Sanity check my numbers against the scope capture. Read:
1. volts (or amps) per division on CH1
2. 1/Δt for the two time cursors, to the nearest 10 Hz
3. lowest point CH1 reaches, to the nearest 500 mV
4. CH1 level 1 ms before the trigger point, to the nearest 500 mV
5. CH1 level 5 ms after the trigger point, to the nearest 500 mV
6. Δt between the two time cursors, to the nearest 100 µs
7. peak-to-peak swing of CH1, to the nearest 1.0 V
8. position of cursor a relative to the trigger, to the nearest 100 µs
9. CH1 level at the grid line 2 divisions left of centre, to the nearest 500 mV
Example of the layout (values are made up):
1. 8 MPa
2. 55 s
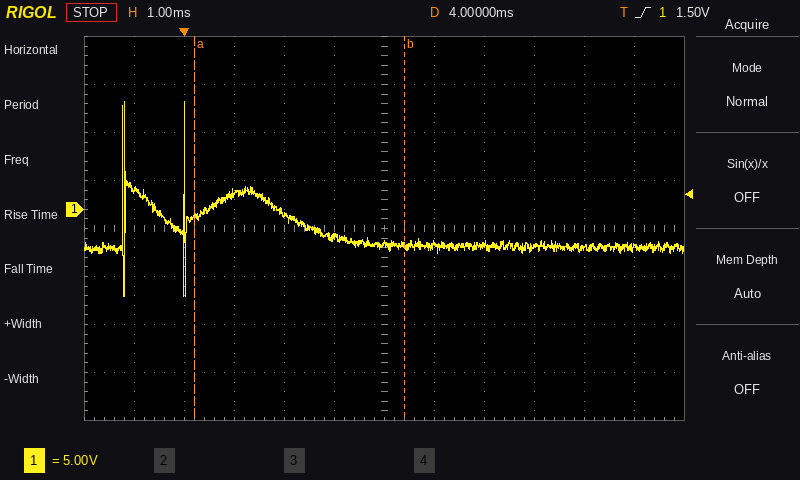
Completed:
1. 5 V
2. 240 Hz
3. -9.0 V
4. 2.0 V
5. -3.5 V
6. 4.2 ms
7. 20.0 V
8. +200 µs
9. -500 mV
